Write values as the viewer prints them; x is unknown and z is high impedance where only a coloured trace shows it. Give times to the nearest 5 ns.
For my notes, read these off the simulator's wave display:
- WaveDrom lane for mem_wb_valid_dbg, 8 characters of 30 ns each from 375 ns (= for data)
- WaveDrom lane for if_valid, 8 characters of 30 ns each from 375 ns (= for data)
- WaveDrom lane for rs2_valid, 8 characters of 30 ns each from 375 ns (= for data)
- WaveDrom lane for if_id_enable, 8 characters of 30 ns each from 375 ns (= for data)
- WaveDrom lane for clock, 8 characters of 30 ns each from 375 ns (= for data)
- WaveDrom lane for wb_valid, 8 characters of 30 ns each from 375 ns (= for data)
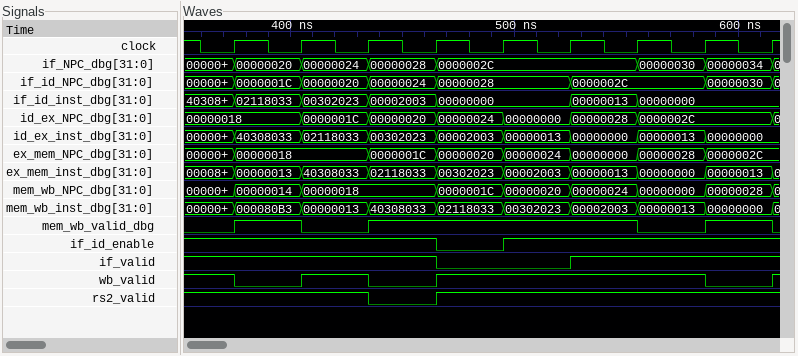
{name: 'mem_wb_valid_dbg', wave: '101...01'}
{name: 'if_valid', wave: '1..0.1..'}
{name: 'rs2_valid', wave: '1.01....'}
{name: 'if_id_enable', wave: '1..01...'}
{name: 'clock', wave: 'p.......'}
{name: 'wb_valid', wave: '0101...0'}
